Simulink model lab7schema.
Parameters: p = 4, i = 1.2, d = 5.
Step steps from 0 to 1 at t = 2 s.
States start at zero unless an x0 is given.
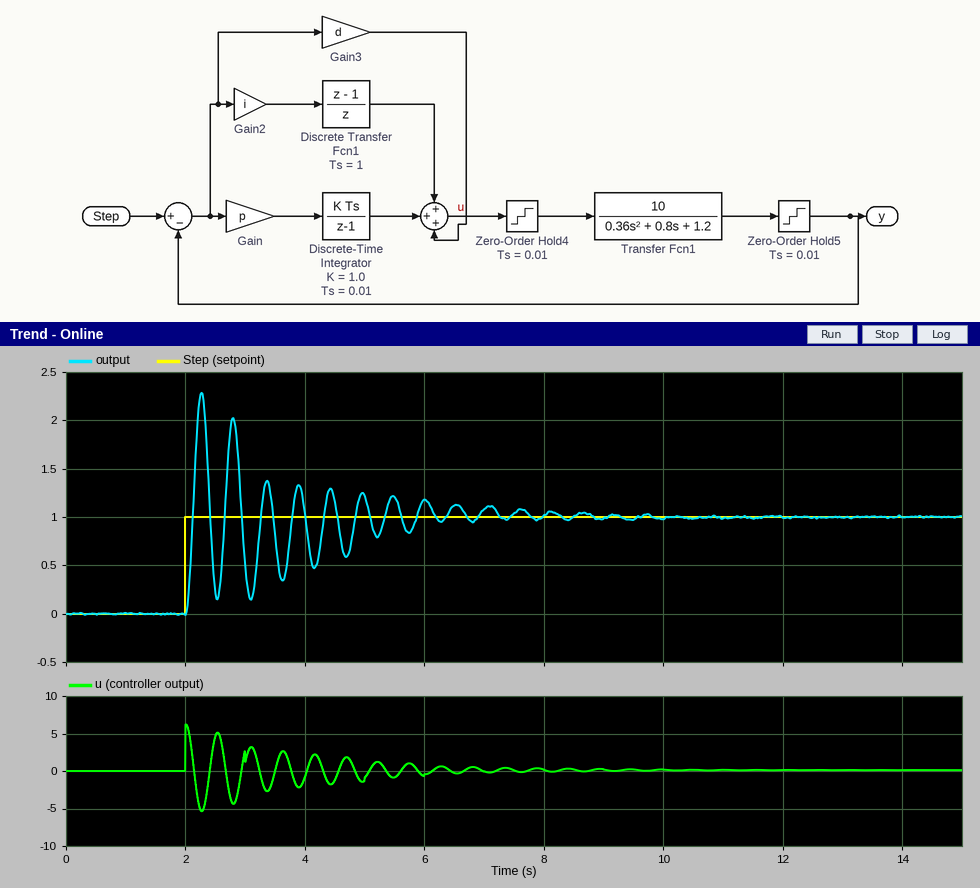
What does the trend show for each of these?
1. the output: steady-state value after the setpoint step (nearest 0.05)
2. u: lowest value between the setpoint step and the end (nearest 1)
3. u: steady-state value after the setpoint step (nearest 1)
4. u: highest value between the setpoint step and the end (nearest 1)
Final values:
1.00
-5
0
6
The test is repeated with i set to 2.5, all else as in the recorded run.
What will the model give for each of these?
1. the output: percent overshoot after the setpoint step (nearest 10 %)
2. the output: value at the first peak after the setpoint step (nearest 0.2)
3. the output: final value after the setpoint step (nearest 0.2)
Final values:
170 %
2.8
1.0
